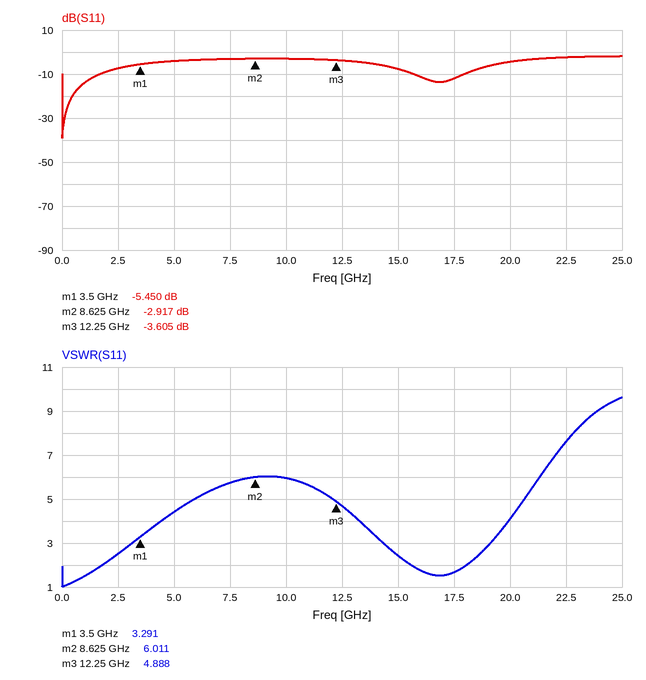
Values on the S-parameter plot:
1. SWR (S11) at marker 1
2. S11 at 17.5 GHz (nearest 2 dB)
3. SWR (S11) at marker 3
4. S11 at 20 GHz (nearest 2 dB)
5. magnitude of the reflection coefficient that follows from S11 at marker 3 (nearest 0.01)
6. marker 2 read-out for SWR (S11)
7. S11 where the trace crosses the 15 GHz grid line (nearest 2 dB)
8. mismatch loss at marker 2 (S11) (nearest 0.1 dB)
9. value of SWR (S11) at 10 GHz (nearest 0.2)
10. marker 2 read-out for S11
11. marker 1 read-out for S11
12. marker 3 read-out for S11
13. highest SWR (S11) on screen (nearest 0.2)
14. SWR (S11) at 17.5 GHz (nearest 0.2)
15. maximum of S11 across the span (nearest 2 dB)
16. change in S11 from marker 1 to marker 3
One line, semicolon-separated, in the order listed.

3.291; -12 dB; 4.888; -4 dB; 0.66; 6.011; -8 dB; 3.1 dB; 6.0; -2.917 dB; -5.450 dB; -3.605 dB; 9.6; 1.6; -2 dB; 1.845 dB
